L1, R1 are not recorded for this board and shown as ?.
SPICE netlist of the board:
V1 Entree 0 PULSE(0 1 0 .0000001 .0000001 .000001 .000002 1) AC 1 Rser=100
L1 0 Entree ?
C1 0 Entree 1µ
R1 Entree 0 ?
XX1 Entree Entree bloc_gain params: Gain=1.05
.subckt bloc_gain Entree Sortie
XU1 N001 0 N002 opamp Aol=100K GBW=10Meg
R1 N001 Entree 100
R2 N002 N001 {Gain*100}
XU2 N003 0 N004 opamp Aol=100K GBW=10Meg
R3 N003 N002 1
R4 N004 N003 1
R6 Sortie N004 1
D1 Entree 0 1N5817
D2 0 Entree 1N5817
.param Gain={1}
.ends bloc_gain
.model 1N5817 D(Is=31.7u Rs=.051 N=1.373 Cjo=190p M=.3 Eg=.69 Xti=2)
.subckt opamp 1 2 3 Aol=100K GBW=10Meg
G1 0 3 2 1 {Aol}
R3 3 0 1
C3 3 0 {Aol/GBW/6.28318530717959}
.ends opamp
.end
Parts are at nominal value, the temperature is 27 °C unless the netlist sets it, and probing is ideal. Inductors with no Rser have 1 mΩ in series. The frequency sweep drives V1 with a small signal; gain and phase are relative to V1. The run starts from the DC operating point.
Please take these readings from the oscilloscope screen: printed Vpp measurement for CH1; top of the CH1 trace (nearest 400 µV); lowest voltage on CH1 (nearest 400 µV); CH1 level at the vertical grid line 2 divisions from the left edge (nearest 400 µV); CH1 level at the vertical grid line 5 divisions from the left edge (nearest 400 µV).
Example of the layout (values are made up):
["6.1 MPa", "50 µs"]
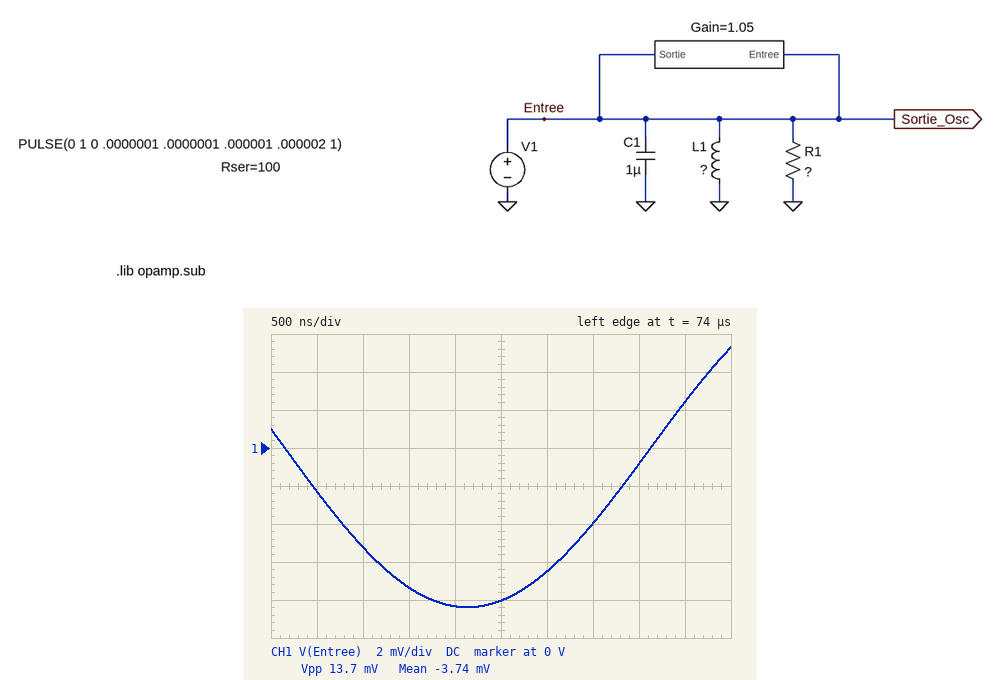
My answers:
["13.7 mV", "5.2 mV", "-8.4 mV", "-5.2 mV", "-8.0 mV"]
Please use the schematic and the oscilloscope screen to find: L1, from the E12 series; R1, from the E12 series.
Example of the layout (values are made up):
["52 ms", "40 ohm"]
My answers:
["1.5 µH", "33 Ω"]
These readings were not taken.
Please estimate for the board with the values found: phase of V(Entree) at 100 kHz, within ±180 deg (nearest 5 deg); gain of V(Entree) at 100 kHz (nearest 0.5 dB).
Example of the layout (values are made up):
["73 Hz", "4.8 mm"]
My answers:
["90 deg", "-32.0 dB"]
